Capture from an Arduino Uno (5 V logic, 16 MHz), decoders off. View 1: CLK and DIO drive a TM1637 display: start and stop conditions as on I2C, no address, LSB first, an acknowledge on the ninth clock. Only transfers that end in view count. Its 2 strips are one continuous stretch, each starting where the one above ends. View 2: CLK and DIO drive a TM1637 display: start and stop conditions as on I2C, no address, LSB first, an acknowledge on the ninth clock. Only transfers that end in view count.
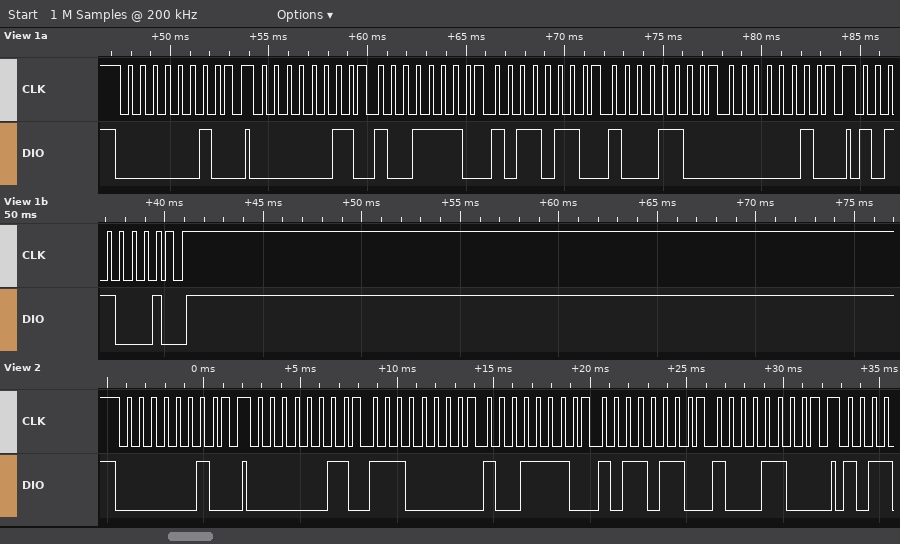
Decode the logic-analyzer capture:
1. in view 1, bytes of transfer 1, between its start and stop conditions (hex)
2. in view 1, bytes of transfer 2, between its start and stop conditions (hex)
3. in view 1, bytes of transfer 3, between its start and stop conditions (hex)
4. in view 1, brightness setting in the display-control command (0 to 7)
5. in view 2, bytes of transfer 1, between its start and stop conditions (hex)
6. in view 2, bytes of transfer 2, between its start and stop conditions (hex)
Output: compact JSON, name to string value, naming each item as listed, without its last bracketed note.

{"in view 1, bytes of transfer 1, between its start and stop conditions": "40", "in view 1, bytes of transfer 2, between its start and stop conditions": "C0 79 6D 31 40", "in view 1, bytes of transfer 3, between its start and stop conditions": "8D", "in view 1, brightness setting in the display-control command": "5", "in view 2, bytes of transfer 1, between its start and stop conditions": "40", "in view 2, bytes of transfer 2, between its start and stop conditions": "C0 07 79 6D 31"}
